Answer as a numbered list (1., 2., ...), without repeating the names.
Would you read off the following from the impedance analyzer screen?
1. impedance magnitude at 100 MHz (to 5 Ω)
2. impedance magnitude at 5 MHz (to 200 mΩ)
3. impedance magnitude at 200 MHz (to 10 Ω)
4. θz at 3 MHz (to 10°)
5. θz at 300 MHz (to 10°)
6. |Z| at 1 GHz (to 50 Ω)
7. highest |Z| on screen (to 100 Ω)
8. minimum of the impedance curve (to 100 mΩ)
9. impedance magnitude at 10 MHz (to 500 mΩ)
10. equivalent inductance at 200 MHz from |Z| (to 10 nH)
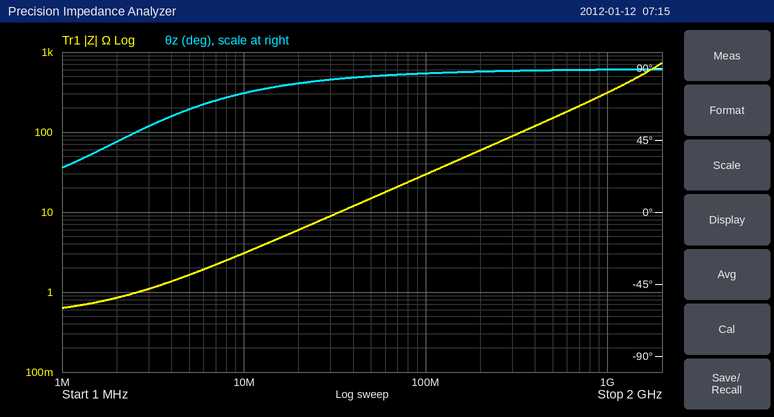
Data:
1. 30 Ω
2. 1.6 Ω
3. 60 Ω
4. 50°
5. 90°
6. 300 Ω
7. 700 Ω
8. 600 mΩ
9. 3.0 Ω
10. 50 nH
